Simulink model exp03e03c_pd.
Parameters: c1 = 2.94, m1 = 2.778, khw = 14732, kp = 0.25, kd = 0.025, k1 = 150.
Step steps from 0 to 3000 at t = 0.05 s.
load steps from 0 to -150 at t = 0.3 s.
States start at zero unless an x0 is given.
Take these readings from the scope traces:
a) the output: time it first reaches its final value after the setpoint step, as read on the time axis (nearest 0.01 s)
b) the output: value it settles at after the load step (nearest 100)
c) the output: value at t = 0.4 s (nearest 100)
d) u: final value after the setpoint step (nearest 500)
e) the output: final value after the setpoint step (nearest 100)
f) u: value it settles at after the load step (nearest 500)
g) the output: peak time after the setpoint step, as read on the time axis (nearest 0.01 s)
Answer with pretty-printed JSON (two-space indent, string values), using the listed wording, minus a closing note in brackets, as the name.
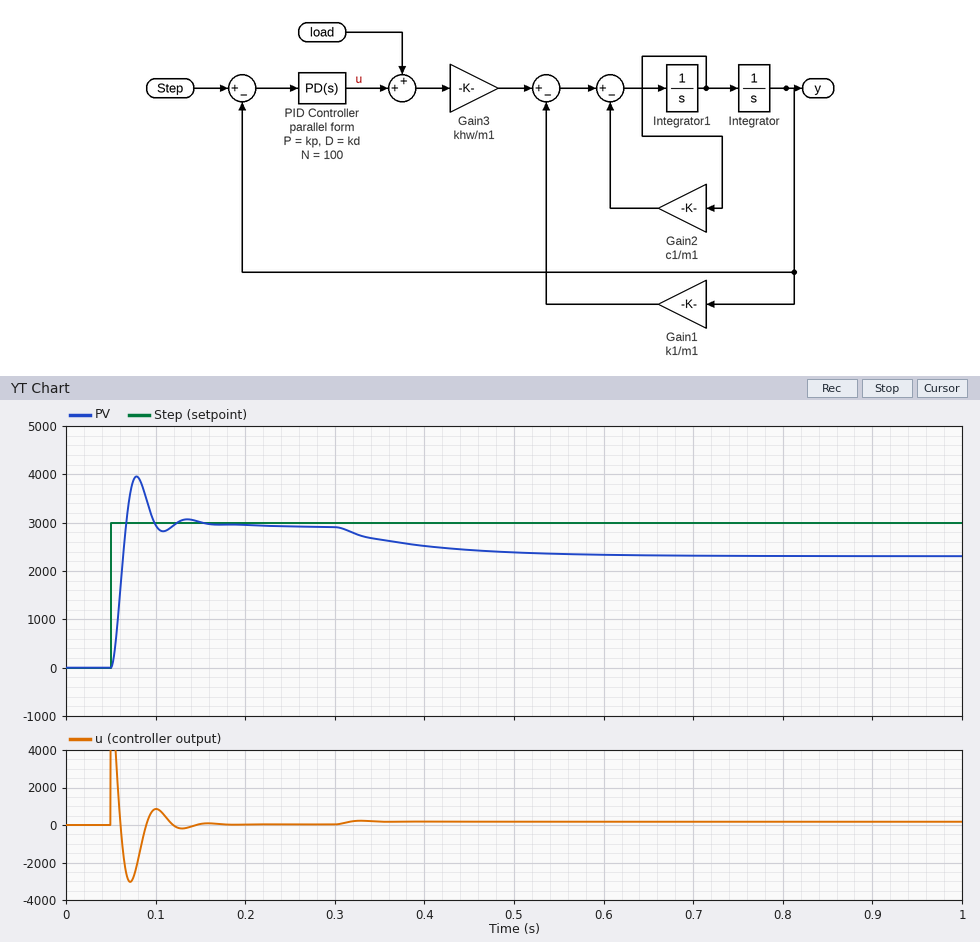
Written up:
{
  "the output: time it first reaches its final value after the setpoint step, as read on the time axis": "0.07 s",
  "the output: value it settles at after the load step": "2300",
  "the output: value at t = 0.4 s": "2500",
  "u: final value after the setpoint step": "0",
  "the output: final value after the setpoint step": "2900",
  "u: value it settles at after the load step": "0",
  "the output: peak time after the setpoint step, as read on the time axis": "0.08 s"
}
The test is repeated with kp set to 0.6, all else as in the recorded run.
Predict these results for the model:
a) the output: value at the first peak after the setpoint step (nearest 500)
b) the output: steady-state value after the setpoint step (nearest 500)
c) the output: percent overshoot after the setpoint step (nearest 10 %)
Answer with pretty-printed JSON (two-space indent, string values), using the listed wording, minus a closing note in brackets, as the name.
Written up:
{
  "the output: value at the first peak after the setpoint step": "4500",
  "the output: steady-state value after the setpoint step": "3000",
  "the output: percent overshoot after the setpoint step": "50 %"
}
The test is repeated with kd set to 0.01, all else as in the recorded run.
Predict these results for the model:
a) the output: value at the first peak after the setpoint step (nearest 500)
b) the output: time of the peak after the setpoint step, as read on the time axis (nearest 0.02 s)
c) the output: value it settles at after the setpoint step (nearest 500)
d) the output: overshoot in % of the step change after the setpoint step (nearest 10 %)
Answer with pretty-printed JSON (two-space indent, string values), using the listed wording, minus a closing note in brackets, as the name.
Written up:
{
  "the output: value at the first peak after the setpoint step": "4000",
  "the output: time of the peak after the setpoint step, as read on the time axis": "0.10 s",
  "the output: value it settles at after the setpoint step": "3000",
  "the output: overshoot in % of the step change after the setpoint step": "40 %"
}
